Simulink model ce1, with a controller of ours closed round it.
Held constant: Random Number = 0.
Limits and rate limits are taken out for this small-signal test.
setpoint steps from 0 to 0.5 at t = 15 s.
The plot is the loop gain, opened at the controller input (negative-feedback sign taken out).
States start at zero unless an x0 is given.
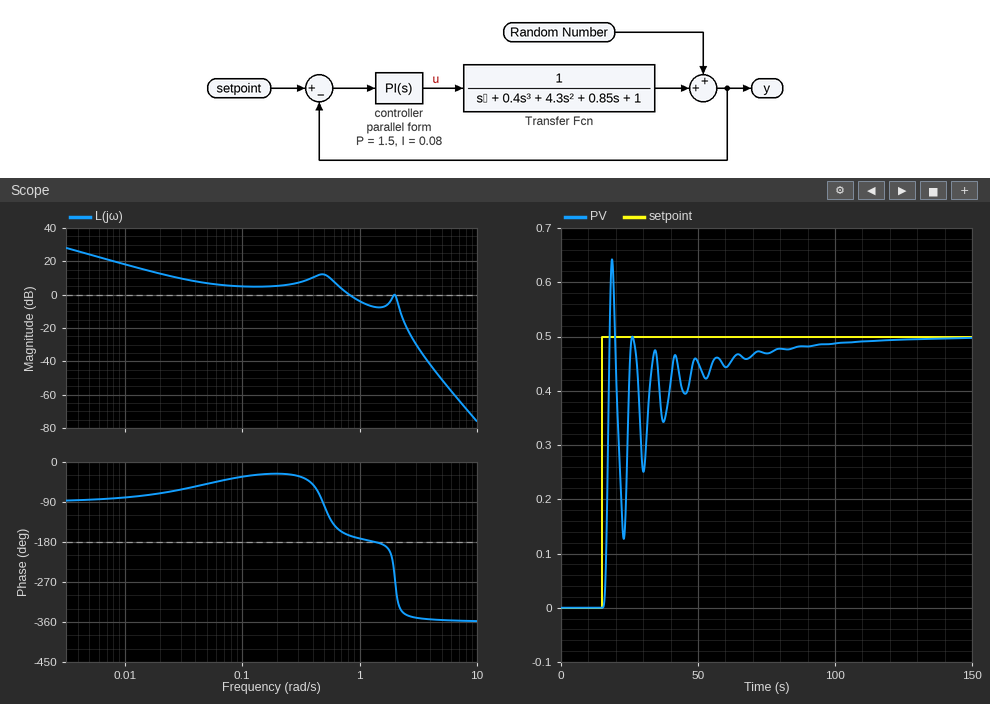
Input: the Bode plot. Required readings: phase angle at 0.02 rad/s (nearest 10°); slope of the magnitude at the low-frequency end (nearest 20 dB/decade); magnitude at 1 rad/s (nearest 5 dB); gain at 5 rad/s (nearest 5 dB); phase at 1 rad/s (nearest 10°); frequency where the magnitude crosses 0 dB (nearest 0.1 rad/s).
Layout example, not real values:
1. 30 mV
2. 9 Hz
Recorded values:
1. -70°
2. -20 dB/decade
3. -5 dB
4. -50 dB
5. -170°
6. 0.8 rad/s
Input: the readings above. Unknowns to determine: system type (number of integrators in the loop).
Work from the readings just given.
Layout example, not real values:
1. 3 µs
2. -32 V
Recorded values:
1. 1
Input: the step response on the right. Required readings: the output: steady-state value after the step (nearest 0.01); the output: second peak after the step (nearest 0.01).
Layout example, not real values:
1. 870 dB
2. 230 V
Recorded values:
1. 0.50
2. 0.50
